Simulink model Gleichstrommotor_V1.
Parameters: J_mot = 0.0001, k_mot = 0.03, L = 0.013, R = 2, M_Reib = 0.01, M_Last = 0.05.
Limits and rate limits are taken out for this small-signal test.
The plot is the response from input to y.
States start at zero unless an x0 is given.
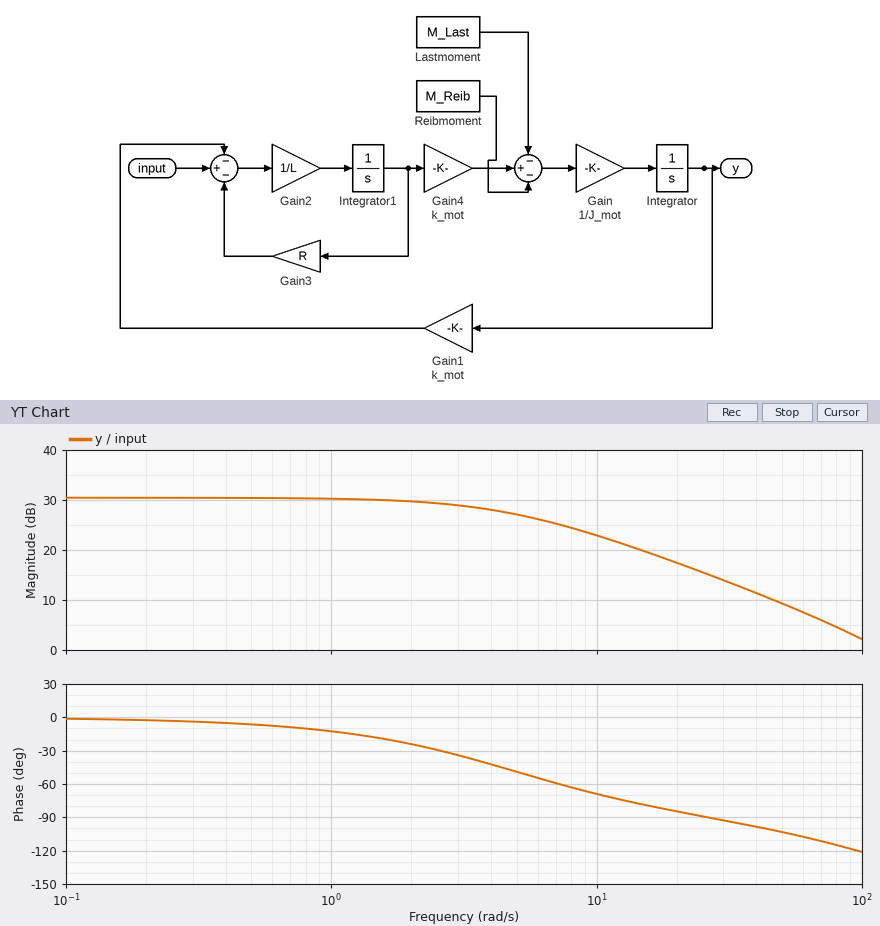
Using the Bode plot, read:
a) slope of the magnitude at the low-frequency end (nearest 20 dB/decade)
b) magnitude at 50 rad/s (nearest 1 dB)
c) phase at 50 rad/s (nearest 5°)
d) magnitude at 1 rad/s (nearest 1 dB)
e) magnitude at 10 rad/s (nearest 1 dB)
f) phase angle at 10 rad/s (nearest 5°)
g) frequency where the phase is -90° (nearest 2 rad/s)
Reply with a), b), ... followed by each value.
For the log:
a) 0 dB/decade
b) 9 dB
c) -105°
d) 30 dB
e) 23 dB
f) -70°
g) 26 rad/s
